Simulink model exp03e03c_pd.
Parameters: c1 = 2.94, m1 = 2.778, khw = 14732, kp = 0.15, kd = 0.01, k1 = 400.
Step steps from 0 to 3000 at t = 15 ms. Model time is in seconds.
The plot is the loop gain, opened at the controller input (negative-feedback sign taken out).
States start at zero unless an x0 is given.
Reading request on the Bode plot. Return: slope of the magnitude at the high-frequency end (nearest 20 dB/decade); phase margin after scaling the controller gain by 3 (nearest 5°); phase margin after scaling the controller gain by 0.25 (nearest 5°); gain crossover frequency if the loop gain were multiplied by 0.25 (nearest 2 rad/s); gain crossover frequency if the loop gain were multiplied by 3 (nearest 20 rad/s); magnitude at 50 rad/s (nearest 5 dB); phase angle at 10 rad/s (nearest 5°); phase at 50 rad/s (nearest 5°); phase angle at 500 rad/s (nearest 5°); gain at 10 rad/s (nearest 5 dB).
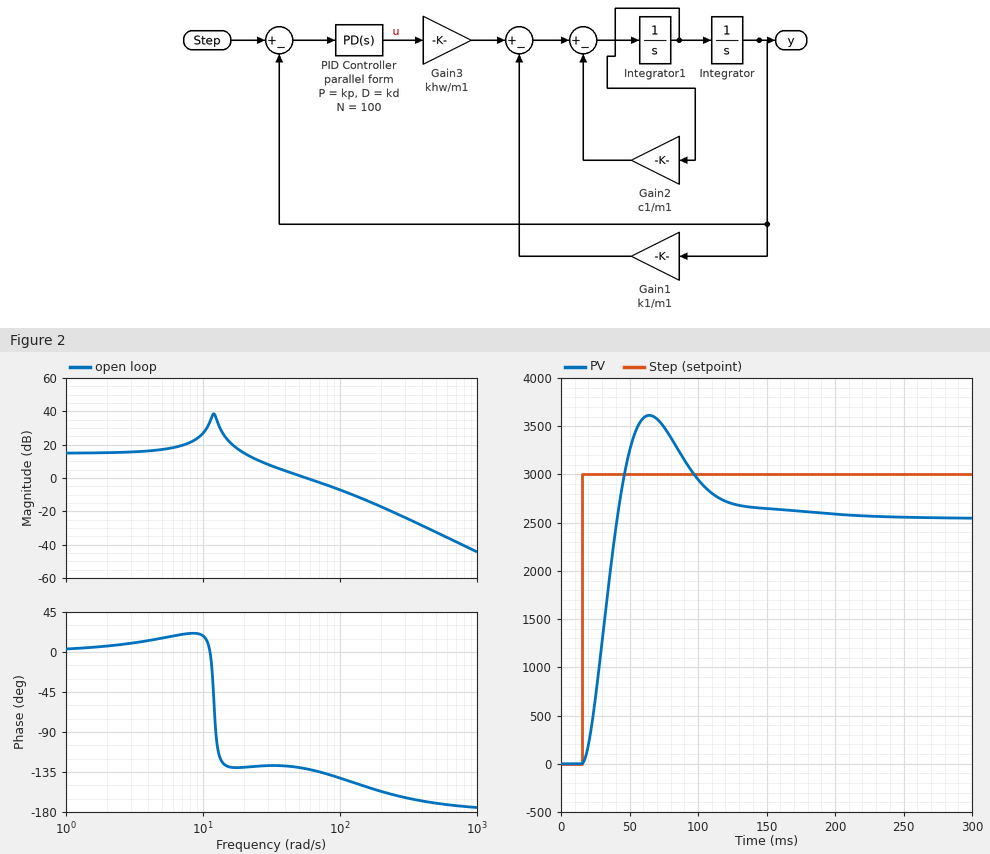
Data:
-40 dB/decade
35°
50°
24 rad/s
120 rad/s
0 dB
20°
-130°
-170°
25 dB
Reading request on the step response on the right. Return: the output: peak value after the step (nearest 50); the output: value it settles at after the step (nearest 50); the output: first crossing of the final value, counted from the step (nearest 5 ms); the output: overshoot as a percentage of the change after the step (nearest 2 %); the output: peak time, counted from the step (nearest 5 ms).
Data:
3600
2550
25 ms
42 %
50 ms
